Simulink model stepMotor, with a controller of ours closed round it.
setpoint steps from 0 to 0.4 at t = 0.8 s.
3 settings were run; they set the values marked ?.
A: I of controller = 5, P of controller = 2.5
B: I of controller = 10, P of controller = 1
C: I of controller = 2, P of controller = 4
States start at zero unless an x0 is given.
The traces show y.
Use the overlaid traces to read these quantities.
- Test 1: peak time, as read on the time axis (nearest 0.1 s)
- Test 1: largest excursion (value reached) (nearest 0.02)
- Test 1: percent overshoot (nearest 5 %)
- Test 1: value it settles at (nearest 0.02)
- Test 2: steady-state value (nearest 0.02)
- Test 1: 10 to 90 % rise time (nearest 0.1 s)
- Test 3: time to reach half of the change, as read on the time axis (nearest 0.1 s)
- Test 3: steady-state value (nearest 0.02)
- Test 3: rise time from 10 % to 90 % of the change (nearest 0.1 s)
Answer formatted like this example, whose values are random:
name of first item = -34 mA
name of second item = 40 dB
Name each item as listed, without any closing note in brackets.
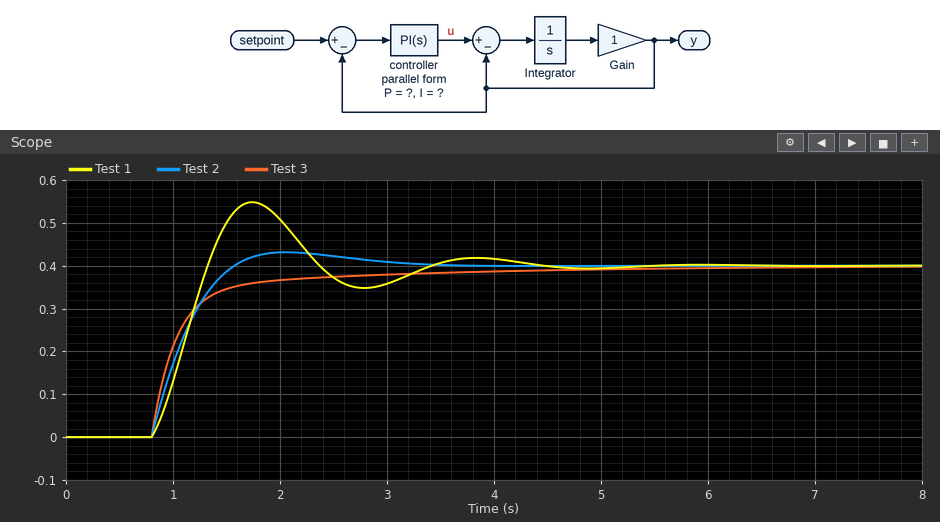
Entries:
Test 1: peak time, as read on the time axis = 1.7 s
Test 1: largest excursion (value reached) = 0.54
Test 1: percent overshoot = 35 %
Test 1: value it settles at = 0.40
Test 2: steady-state value = 0.40
Test 1: 10 to 90 % rise time = 0.4 s
Test 3: time to reach half of the change, as read on the time axis = 1.0 s
Test 3: steady-state value = 0.40
Test 3: rise time from 10 % to 90 % of the change = 0.9 s
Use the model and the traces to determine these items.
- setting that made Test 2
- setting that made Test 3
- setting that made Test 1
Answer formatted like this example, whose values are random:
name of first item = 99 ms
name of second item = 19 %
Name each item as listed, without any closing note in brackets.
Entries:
setting that made Test 2 = A
setting that made Test 3 = C
setting that made Test 1 = B
